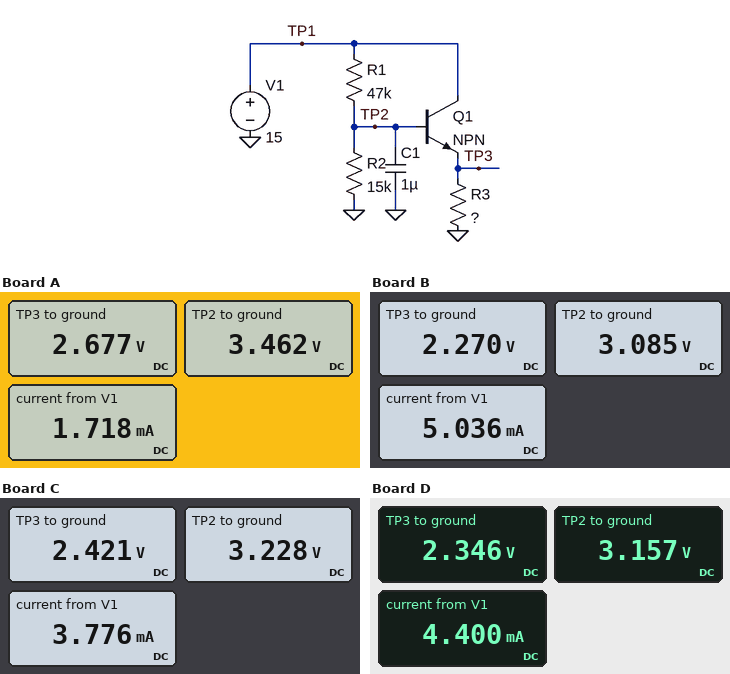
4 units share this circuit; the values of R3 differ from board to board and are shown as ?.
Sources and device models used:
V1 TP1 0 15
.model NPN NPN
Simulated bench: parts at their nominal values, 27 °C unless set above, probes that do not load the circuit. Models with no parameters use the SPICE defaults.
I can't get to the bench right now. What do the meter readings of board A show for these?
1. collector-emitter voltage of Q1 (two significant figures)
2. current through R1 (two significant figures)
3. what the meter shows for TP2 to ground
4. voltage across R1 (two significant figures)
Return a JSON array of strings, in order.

["12 V", "250 µA", "3.462 V", "12 V"]
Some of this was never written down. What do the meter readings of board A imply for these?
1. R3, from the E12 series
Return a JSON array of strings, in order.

["1.8 kΩ"]
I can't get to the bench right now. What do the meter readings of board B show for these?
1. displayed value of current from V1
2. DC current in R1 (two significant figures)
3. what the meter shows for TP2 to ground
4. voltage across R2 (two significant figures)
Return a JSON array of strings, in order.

["5.036 mA", "250 µA", "3.085 V", "3.1 V"]
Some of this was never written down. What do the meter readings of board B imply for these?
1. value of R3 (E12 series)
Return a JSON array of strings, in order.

["470 Ω"]
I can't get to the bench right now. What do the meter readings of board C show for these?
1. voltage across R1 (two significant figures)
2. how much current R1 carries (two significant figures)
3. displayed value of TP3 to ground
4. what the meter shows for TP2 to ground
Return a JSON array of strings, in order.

["12 V", "250 µA", "2.421 V", "3.228 V"]
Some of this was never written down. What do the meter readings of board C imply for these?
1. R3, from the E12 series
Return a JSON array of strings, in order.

["680 Ω"]
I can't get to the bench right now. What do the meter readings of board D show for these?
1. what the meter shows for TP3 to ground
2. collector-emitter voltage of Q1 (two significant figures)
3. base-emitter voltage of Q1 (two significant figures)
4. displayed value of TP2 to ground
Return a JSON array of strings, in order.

["2.346 V", "13 V", "810 mV", "3.157 V"]
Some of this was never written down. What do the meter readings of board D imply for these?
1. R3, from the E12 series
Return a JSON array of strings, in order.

["560 Ω"]
